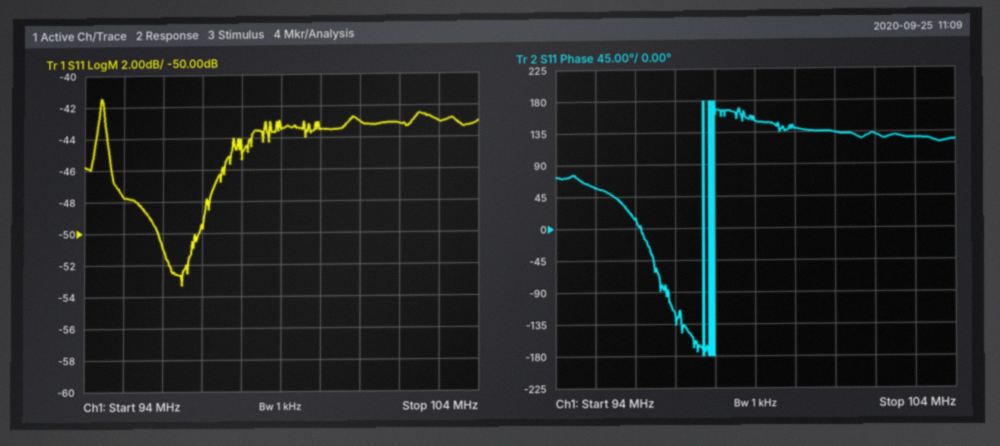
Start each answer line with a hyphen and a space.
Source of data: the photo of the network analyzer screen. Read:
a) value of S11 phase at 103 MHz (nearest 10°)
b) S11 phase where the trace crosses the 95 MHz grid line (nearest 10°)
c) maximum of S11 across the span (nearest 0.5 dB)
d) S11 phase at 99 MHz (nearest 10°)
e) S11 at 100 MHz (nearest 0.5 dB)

- 130°
- 60°
- -41.5 dB
- 150°
- -43.5 dB
